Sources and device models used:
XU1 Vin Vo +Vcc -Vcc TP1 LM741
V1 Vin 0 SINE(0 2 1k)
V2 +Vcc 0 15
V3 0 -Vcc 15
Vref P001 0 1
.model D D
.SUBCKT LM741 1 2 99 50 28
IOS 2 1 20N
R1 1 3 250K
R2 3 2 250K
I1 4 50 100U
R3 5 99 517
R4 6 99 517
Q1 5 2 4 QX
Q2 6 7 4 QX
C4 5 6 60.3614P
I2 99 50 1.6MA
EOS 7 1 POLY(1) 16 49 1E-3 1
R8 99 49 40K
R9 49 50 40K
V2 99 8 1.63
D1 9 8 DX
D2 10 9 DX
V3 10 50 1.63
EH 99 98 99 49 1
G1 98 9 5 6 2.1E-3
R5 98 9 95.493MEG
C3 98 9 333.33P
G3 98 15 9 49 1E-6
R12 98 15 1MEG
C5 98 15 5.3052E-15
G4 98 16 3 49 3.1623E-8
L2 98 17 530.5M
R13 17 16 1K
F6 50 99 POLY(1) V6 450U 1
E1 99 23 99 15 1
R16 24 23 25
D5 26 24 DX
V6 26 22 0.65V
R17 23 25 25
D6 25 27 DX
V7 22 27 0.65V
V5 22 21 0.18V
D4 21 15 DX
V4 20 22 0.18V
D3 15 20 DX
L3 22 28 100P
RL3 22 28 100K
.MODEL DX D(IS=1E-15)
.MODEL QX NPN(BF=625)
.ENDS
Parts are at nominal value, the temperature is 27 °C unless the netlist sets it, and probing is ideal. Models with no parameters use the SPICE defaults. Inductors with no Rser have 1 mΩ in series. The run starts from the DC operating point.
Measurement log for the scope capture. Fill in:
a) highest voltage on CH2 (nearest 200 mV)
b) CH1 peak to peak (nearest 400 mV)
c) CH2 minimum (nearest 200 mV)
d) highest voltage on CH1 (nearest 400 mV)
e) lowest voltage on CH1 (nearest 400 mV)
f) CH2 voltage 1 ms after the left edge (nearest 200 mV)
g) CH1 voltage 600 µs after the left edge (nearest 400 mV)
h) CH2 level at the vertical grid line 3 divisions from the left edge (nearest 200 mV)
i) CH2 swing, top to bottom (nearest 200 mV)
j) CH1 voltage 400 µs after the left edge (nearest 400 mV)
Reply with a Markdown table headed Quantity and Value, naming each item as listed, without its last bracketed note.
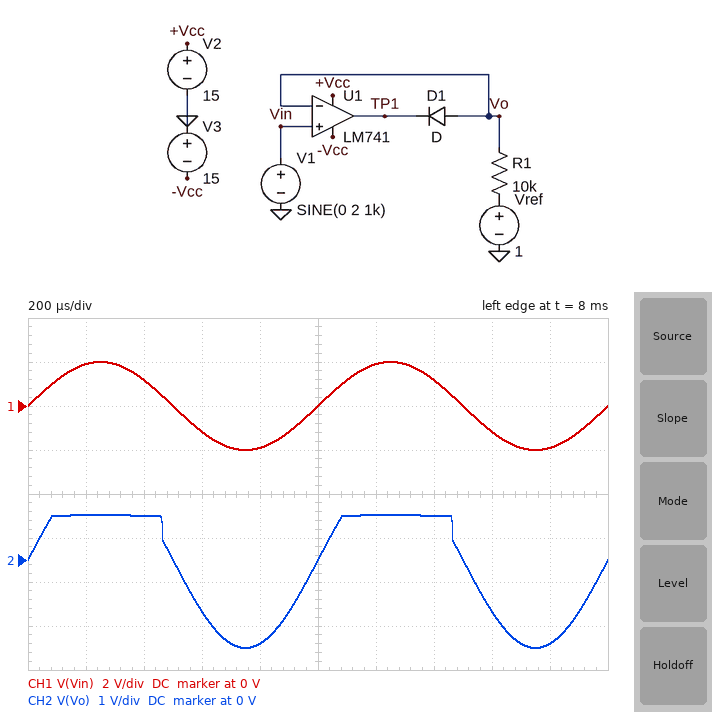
| Quantity | Value |
|---|---|
| highest voltage on CH2 | 1.0 V |
| CH1 peak to peak | 4.0 V |
| CH2 minimum | -2.0 V |
| highest voltage on CH1 | 2.0 V |
| lowest voltage on CH1 | -2.0 V |
| CH2 voltage 1 ms after the left edge | 0 V |
| CH1 voltage 600 µs after the left edge | -1.2 V |
| CH2 level at the vertical grid line 3 divisions from the left edge | -1.2 V |
| CH2 swing, top to bottom | 3.0 V |
| CH1 voltage 400 µs after the left edge | 1.2 V |
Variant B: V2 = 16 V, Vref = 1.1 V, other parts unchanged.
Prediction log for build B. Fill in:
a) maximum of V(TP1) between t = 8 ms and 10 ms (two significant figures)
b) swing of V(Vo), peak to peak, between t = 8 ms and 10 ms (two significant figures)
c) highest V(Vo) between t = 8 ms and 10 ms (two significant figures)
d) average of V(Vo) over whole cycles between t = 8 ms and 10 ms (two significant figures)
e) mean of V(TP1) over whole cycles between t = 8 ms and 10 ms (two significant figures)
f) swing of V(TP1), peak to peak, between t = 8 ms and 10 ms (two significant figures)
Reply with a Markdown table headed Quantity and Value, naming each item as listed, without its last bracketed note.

| Quantity | Value |
|---|---|
| maximum of V(TP1) between t = 8 ms and 10 ms | 15 V |
| swing of V(Vo), peak to peak, between t = 8 ms and 10 ms | 3.1 V |
| highest V(Vo) between t = 8 ms and 10 ms | 1.1 V |
| average of V(Vo) over whole cycles between t = 8 ms and 10 ms | -170 mV |
| mean of V(TP1) over whole cycles between t = 8 ms and 10 ms | 3.8 V |
| swing of V(TP1), peak to peak, between t = 8 ms and 10 ms | 18 V |
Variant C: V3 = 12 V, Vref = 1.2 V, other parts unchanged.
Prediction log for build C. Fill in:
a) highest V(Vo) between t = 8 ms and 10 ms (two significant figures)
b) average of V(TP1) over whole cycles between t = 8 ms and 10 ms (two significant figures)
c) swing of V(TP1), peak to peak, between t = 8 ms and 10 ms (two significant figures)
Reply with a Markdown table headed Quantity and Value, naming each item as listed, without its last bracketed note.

| Quantity | Value |
|---|---|
| highest V(Vo) between t = 8 ms and 10 ms | 1.2 V |
| average of V(TP1) over whole cycles between t = 8 ms and 10 ms | 3.2 V |
| swing of V(TP1), peak to peak, between t = 8 ms and 10 ms | 17 V |
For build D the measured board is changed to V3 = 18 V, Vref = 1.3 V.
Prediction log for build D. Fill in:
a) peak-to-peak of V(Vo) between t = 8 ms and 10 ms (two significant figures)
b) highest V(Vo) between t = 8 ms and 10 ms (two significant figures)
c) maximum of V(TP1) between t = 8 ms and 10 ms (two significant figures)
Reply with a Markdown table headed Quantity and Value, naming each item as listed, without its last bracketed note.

| Quantity | Value |
|---|---|
| peak-to-peak of V(Vo) between t = 8 ms and 10 ms | 3.3 V |
| highest V(Vo) between t = 8 ms and 10 ms | 1.3 V |
| maximum of V(TP1) between t = 8 ms and 10 ms | 14 V |
